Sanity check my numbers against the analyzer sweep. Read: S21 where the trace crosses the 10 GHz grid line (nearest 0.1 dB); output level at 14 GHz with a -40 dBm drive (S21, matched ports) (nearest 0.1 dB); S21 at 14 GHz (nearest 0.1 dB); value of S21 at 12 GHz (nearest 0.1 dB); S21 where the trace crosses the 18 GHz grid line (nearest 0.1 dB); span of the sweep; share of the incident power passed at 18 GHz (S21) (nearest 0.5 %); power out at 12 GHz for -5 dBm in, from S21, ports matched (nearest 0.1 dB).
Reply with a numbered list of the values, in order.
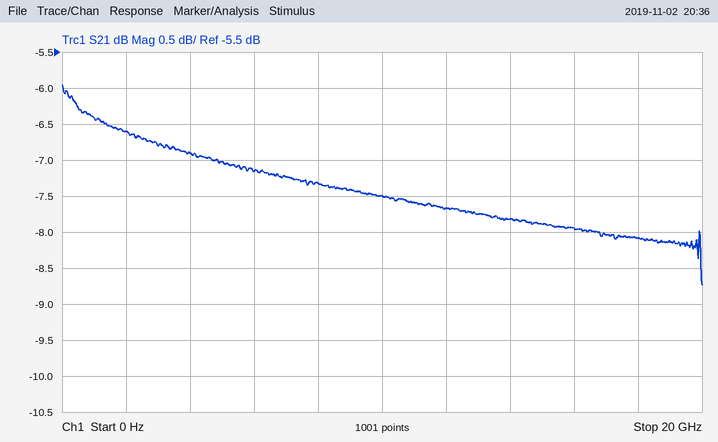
1. -7.5 dB
2. -47.8 dBm
3. -7.8 dB
4. -7.7 dB
5. -8.1 dB
6. 20 GHz
7. 15.5 %
8. -12.7 dBm
